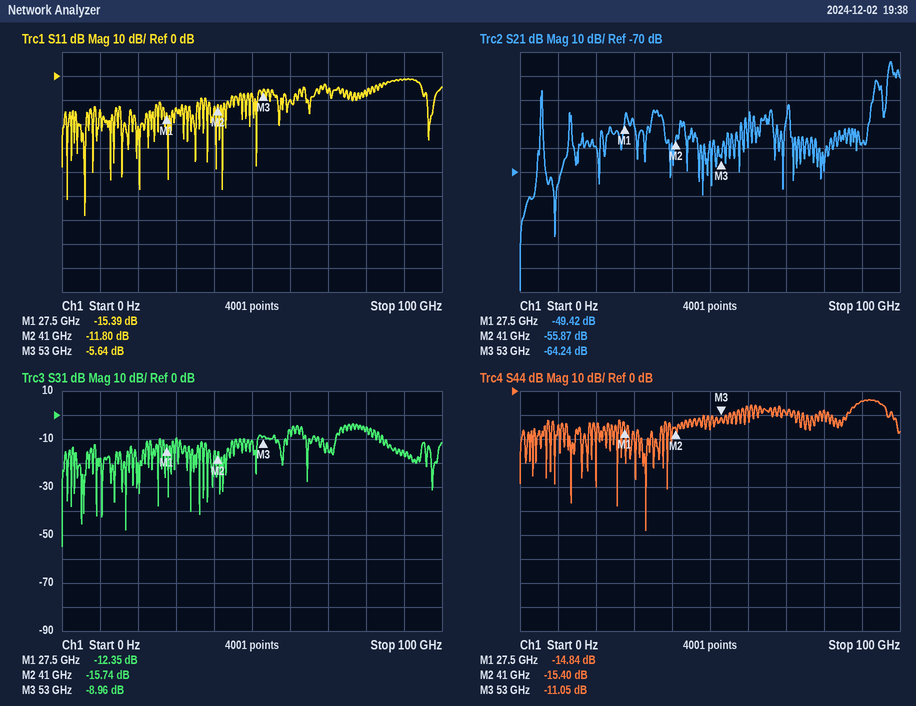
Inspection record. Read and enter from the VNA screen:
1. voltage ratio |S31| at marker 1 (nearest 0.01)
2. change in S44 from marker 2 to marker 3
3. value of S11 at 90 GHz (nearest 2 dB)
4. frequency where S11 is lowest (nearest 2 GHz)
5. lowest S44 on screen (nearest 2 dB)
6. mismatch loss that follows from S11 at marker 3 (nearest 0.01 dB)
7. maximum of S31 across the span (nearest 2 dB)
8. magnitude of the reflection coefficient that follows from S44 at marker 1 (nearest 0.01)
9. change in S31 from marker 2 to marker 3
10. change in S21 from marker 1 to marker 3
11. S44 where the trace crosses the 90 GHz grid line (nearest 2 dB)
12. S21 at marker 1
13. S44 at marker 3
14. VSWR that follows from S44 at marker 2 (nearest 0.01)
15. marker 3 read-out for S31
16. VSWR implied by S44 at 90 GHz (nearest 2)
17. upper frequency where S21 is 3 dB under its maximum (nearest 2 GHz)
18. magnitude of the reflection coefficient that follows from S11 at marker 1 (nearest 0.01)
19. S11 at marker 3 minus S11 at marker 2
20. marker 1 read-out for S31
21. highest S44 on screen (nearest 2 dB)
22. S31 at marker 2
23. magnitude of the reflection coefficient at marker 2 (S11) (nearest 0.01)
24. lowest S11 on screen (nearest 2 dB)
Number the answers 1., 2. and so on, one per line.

1. 0.24
2. 4.35 dB
3. -2 dB
4. 6 GHz
5. -58 dB
6. 1.38 dB
7. -4 dB
8. 0.18
9. 6.78 dB
10. -14.82 dB
11. -4 dB
12. -49.42 dB
13. -11.05 dB
14. 1.41
15. -8.96 dB
16. 4
17. 98 GHz
18. 0.17
19. 6.16 dB
20. -12.35 dB
21. -4 dB
22. -15.74 dB
23. 0.26
24. -58 dB
